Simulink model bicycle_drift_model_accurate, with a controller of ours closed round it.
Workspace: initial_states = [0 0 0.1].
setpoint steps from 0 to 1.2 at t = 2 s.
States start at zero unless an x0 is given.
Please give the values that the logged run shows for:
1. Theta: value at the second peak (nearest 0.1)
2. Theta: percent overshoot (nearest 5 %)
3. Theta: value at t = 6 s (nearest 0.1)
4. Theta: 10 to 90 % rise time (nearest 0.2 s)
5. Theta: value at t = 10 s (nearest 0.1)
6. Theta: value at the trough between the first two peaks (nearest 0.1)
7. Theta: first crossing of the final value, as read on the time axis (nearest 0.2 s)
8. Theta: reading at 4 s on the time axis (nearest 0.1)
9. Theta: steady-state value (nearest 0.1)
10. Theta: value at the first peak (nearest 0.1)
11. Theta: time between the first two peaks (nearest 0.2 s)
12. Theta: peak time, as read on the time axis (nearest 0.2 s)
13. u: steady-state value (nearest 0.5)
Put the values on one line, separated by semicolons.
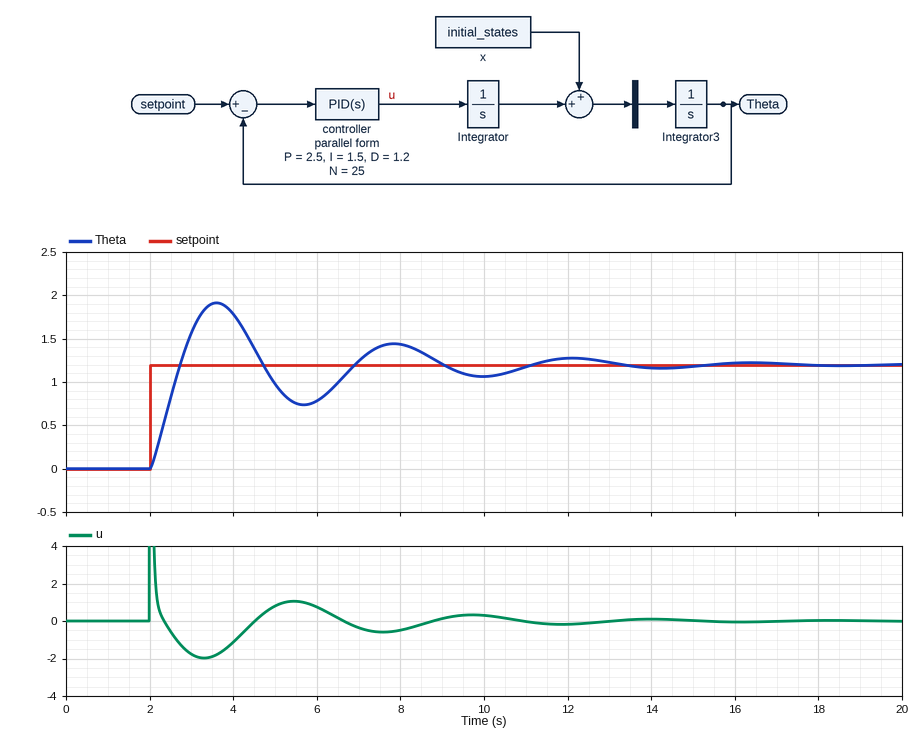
1.4; 60 %; 0.8; 0.6 s; 1.1; 0.7; 2.8 s; 1.8; 1.2; 1.9; 4.2 s; 3.6 s; 0.0
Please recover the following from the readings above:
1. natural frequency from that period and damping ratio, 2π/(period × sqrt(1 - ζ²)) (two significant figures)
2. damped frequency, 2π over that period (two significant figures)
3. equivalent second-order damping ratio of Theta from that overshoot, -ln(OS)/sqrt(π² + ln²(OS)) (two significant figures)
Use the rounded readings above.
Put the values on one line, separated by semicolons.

1.5 rad/s; 1.5 rad/s; 0.16
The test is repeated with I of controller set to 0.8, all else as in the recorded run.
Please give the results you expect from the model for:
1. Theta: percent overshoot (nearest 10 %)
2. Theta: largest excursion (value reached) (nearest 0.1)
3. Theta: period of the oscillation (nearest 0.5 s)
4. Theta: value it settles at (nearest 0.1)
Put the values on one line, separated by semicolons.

50 %; 1.8; 4.5 s; 1.2
